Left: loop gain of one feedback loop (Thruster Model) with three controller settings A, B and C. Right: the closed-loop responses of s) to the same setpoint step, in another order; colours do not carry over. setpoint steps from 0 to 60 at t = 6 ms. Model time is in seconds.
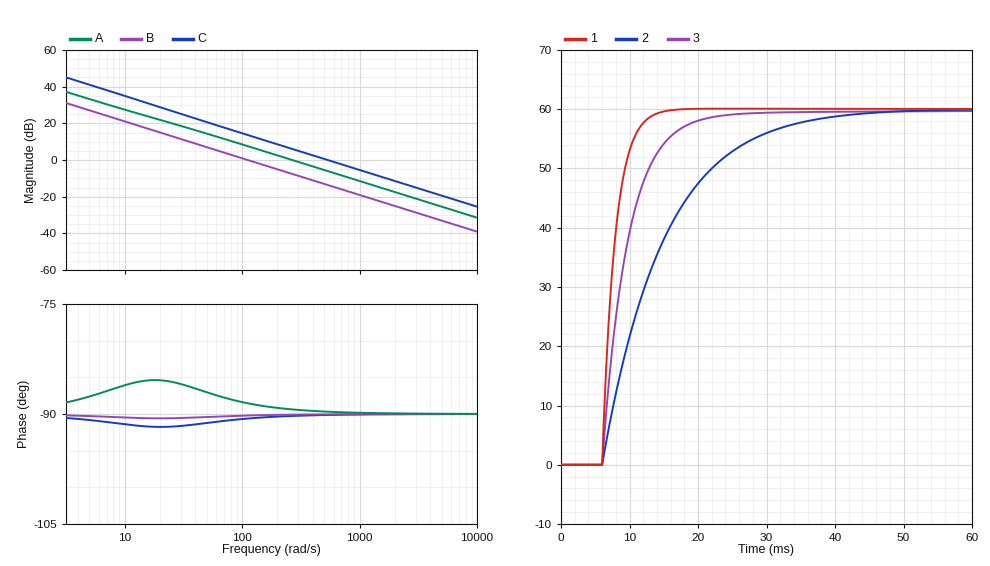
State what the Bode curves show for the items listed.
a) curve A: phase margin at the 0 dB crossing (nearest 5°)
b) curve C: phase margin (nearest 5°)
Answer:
90°
90°
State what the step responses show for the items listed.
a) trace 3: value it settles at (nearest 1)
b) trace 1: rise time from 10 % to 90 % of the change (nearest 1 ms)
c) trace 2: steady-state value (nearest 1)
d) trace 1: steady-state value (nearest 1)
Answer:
60
4 ms
60
60
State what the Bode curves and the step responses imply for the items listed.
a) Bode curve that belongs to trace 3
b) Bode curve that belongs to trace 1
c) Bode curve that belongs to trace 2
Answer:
A
C
B
